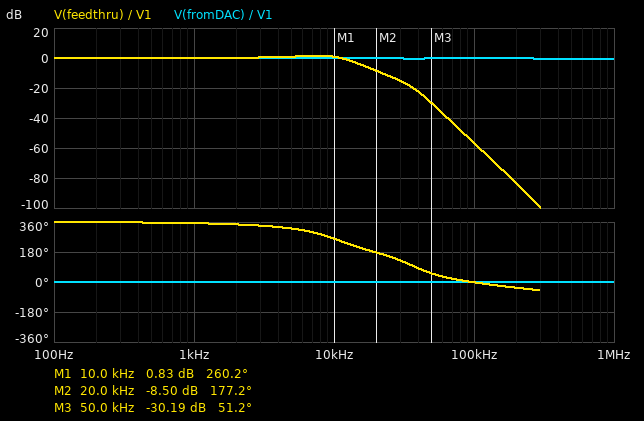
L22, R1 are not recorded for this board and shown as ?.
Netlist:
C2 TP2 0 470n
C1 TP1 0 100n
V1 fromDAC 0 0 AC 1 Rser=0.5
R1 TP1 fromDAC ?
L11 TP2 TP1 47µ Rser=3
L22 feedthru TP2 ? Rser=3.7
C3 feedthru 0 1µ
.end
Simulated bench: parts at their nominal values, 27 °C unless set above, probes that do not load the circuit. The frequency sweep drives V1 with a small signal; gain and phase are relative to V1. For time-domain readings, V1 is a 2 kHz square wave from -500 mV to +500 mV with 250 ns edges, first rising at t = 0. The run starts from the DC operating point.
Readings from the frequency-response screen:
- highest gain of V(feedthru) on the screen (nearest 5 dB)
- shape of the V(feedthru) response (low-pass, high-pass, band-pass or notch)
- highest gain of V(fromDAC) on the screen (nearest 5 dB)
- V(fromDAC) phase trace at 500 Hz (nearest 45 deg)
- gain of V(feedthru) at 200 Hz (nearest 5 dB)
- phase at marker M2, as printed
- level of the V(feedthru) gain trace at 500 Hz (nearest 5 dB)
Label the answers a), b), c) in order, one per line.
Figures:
a) 0 dB
b) low-pass
c) 0 dB
d) 0 deg
e) 0 dB
f) 177.2 deg
g) 0 dB
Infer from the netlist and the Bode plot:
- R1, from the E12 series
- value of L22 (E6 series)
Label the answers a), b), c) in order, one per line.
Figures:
a) 6.8 Ω
b) 220 µH
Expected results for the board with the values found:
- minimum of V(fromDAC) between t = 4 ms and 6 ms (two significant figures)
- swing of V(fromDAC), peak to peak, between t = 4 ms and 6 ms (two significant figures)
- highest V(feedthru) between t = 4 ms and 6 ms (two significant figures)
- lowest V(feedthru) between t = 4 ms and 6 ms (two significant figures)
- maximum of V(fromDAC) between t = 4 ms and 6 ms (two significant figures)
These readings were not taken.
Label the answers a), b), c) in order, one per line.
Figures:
a) -500 mV
b) 1.0 V
c) 670 mV
d) -670 mV
e) 500 mV
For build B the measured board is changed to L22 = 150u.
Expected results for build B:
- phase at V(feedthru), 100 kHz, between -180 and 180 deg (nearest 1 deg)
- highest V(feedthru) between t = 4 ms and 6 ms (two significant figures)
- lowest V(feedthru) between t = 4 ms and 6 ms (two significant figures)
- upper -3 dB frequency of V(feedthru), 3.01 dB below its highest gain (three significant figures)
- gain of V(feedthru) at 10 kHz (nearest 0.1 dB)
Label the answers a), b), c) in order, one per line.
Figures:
a) -1 deg
b) 600 mV
c) -600 mV
d) 14.8 kHz
e) 0 dB
